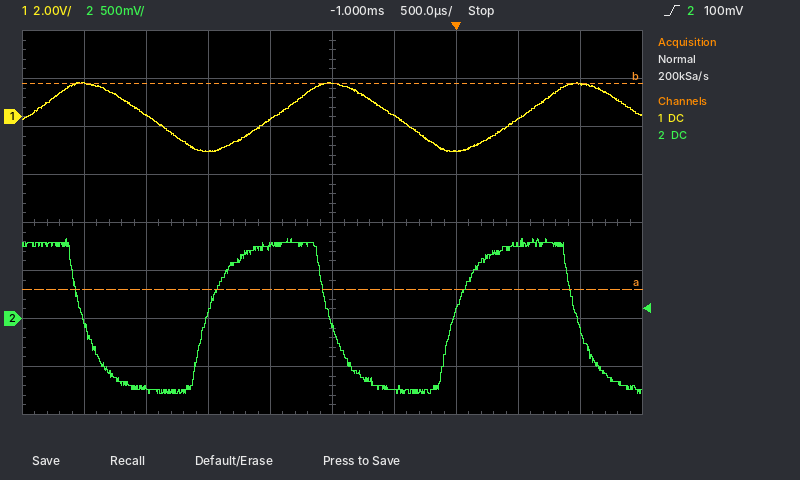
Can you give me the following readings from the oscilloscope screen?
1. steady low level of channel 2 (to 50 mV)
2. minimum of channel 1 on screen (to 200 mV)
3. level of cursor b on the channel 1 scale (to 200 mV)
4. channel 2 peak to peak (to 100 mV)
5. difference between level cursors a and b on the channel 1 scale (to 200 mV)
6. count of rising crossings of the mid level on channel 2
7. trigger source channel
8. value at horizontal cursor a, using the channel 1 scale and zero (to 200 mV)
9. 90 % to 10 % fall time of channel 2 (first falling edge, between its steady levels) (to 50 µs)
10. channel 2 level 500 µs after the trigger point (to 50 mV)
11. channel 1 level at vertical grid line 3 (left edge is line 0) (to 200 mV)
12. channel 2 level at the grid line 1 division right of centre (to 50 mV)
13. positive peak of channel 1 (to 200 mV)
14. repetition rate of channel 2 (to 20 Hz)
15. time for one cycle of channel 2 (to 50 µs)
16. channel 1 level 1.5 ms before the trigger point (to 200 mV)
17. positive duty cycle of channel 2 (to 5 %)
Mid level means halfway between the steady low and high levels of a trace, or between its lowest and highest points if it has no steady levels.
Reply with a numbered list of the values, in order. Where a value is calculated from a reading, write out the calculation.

1. -750 mV
2. -1.4 V
3. 1.4 V
4. 1.60 V
5. 8.6 V
6. 2
7. channel 2
8. -7.2 V
9. 350 µs
10. 800 mV
11. -1.4 V
12. -750 mV
13. 1.4 V
14. 1 / 2.00 ms ≈ 500 Hz
15. 2.00 ms
16. -200 mV
17. 50 %
